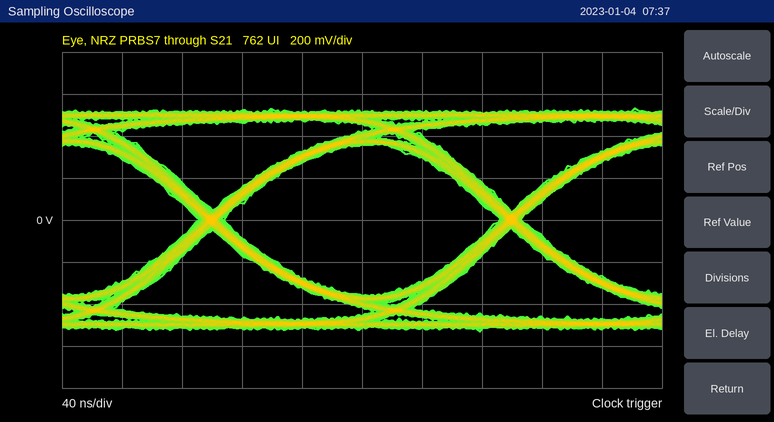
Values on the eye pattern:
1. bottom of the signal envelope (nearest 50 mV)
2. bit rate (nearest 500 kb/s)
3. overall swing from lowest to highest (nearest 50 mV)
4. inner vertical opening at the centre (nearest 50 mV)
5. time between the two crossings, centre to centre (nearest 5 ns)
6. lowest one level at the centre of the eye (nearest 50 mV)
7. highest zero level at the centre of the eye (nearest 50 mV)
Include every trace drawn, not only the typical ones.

-550 mV
5.0 Mb/s
1.05 V
700 mV
200 ns
350 mV
-350 mV
